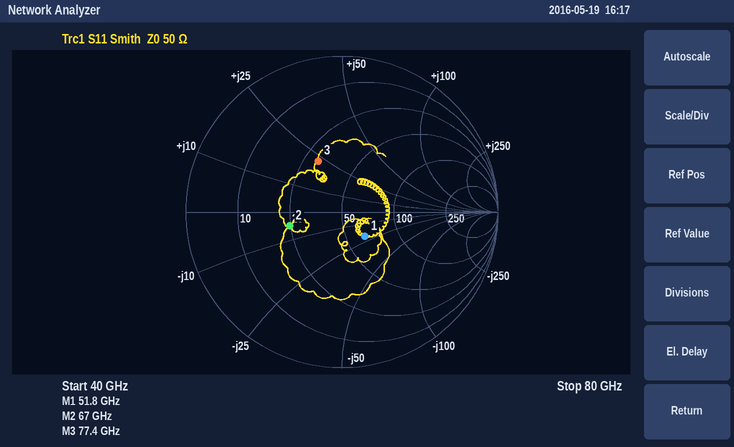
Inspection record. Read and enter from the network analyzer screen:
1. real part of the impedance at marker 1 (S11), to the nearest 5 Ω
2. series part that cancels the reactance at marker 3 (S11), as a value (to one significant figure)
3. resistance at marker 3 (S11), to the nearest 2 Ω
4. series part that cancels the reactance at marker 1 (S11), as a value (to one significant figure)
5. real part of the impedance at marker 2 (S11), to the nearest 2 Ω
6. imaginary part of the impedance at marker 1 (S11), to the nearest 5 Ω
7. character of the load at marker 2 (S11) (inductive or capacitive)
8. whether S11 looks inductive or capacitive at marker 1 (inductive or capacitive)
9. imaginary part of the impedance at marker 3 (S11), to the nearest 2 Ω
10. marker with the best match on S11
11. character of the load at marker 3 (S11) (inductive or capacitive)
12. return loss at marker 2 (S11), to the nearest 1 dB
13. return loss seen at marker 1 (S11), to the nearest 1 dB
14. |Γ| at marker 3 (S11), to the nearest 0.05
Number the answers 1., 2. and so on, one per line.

1. 65 Ω
2. 90 fF
3. 30 Ω
4. 60 pH
5. 24 Ω
6. -20 Ω
7. capacitive
8. capacitive
9. +22 Ω
10. marker 1
11. inductive
12. 9 dB
13. 13 dB
14. 0.35
